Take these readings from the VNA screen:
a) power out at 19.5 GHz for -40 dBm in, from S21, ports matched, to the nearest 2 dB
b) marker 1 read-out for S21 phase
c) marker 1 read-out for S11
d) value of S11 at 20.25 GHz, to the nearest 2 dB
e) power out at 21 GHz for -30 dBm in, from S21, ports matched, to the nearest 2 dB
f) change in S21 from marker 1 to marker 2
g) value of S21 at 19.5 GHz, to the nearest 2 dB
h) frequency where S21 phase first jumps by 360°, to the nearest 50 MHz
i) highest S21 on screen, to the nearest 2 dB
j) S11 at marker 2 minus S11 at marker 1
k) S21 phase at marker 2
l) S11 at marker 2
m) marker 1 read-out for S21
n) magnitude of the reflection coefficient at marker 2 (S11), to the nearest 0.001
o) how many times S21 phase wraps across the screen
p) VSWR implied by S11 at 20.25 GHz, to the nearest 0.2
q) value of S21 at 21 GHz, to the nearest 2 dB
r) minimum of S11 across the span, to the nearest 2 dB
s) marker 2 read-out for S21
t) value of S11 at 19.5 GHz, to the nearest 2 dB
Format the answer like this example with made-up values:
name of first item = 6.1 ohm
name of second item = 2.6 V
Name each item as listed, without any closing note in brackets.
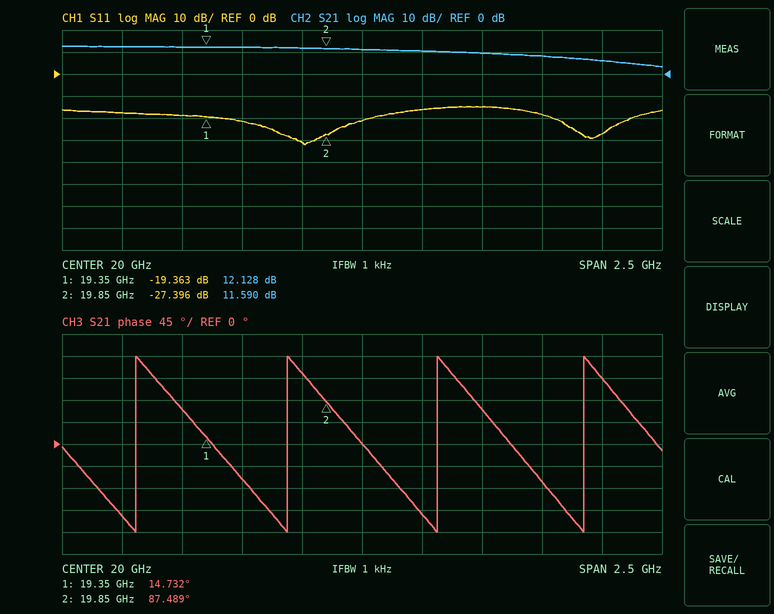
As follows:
power out at 19.5 GHz for -40 dBm in, from S21, ports matched, to the nearest 2 dB = -28 dBm
marker 1 read-out for S21 phase = 14.732°
marker 1 read-out for S11 = -19.363 dB
value of S11 at 20.25 GHz, to the nearest 2 dB = -16 dB
power out at 21 GHz for -30 dBm in, from S21, ports matched, to the nearest 2 dB = -24 dBm
change in S21 from marker 1 to marker 2 = -0.538 dB
value of S21 at 19.5 GHz, to the nearest 2 dB = 12 dB
frequency where S21 phase first jumps by 360°, to the nearest 50 MHz = 19.05 GHz
highest S21 on screen, to the nearest 2 dB = 12 dB
S11 at marker 2 minus S11 at marker 1 = -8.033 dB
S21 phase at marker 2 = 87.489°
S11 at marker 2 = -27.396 dB
marker 1 read-out for S21 = 12.128 dB
magnitude of the reflection coefficient at marker 2 (S11), to the nearest 0.001 = 0.043
how many times S21 phase wraps across the screen = 4
VSWR implied by S11 at 20.25 GHz, to the nearest 0.2 = 1.4
value of S21 at 21 GHz, to the nearest 2 dB = 6 dB
minimum of S11 across the span, to the nearest 2 dB = -32 dB
marker 2 read-out for S21 = 11.590 dB
value of S11 at 19.5 GHz, to the nearest 2 dB = -22 dB
